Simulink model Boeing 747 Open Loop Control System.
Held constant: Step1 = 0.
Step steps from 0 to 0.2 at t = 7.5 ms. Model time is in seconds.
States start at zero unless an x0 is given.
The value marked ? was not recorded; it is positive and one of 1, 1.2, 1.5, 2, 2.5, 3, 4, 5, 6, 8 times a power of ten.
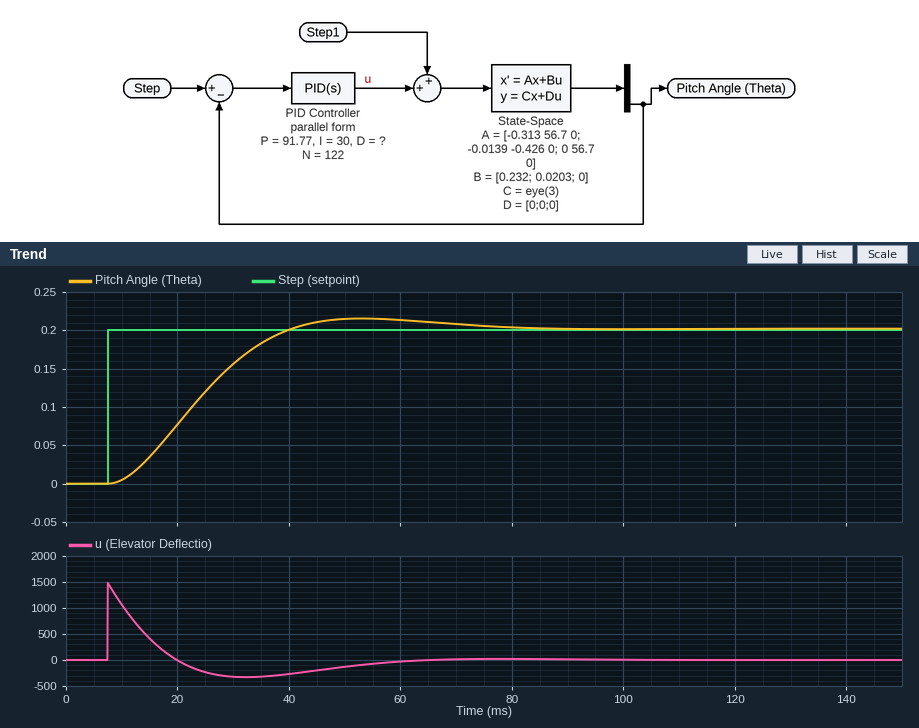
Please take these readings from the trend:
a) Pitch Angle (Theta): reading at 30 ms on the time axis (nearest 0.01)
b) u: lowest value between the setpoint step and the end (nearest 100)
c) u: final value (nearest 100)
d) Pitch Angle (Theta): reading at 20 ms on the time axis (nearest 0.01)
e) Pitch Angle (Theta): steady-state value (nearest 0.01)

0.16
-300
0
0.08
0.20
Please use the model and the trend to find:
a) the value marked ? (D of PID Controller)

60
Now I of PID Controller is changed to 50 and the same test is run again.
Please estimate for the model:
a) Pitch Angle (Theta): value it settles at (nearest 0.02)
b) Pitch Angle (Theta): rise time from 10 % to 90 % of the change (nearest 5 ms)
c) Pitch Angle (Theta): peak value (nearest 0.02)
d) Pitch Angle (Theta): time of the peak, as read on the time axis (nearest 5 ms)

0.20
20 ms
0.22
55 ms
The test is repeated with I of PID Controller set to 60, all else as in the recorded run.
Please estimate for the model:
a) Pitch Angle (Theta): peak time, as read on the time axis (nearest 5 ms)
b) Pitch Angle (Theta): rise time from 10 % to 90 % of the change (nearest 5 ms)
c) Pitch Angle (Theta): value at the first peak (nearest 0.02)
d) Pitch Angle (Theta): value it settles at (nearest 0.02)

55 ms
20 ms
0.22
0.20
